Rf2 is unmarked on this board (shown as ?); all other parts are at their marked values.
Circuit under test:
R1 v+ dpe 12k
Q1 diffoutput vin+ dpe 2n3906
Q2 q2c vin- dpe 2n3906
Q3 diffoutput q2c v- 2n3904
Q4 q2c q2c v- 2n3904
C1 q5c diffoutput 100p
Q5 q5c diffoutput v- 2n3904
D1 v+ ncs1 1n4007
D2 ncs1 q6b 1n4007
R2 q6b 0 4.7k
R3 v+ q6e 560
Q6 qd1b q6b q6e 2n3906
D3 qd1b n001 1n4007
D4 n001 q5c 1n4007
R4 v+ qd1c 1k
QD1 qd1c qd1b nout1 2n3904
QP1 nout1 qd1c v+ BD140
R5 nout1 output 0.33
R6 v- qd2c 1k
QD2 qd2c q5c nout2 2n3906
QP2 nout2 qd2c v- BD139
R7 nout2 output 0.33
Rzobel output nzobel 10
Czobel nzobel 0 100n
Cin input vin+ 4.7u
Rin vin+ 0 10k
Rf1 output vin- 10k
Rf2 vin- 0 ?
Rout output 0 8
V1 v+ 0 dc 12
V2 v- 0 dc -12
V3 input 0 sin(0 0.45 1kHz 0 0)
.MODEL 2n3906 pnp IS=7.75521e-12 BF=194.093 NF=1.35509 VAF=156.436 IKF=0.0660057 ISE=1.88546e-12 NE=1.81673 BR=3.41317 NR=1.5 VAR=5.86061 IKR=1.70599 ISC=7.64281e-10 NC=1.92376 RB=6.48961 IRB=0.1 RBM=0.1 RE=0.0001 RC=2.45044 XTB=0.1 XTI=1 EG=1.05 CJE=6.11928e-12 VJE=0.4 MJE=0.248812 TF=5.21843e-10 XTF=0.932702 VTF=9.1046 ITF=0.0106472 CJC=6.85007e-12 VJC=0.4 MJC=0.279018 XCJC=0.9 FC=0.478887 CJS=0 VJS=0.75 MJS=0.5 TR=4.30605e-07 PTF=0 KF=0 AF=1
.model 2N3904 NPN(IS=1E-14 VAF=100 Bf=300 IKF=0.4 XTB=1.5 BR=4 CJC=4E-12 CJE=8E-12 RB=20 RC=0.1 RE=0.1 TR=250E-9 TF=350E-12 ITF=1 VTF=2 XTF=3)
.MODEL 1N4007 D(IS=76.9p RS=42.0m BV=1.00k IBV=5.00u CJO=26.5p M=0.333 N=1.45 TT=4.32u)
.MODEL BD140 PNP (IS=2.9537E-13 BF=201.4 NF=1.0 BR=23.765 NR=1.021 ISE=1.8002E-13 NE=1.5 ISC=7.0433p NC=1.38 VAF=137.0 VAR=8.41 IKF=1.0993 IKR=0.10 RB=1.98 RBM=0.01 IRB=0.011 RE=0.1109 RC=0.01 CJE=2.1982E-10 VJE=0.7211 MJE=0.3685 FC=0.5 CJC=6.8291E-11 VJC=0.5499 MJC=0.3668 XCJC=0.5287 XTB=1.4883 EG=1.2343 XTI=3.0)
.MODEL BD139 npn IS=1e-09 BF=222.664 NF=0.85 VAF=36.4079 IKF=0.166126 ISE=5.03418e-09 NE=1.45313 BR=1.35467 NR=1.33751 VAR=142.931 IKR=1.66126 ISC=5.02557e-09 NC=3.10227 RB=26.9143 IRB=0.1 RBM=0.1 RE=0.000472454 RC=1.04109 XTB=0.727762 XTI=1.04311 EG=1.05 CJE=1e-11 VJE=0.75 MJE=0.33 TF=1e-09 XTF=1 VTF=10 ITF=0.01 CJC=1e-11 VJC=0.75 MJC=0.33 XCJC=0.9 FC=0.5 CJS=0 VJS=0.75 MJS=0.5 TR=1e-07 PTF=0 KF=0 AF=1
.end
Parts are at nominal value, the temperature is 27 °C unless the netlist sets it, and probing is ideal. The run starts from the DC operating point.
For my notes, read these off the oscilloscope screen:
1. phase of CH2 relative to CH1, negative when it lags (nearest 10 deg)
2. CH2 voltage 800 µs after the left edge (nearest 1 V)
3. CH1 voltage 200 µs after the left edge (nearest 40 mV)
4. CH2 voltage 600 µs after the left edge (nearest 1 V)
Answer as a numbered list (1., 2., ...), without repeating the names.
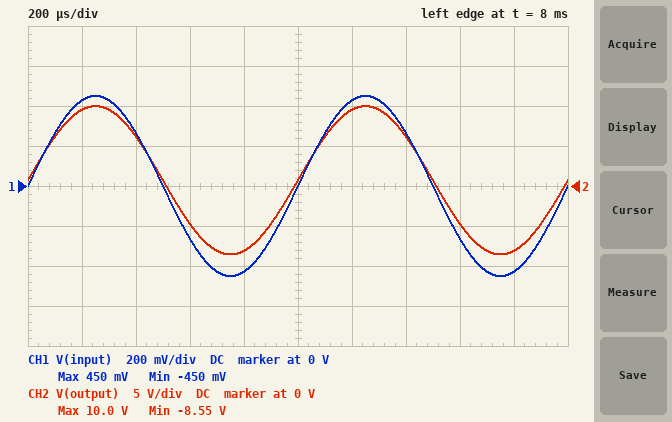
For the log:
1. 0 deg
2. -8 V
3. 440 mV
4. -5 V
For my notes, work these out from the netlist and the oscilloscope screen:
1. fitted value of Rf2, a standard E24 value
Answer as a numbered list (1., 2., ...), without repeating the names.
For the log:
1. 510 Ω
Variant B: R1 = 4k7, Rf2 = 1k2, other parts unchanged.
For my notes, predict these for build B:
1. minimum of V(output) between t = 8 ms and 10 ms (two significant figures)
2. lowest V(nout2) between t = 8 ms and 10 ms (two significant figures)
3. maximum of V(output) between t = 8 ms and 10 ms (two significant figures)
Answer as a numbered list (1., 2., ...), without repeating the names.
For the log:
1. -3.5 V
2. -3.6 V
3. 4.9 V
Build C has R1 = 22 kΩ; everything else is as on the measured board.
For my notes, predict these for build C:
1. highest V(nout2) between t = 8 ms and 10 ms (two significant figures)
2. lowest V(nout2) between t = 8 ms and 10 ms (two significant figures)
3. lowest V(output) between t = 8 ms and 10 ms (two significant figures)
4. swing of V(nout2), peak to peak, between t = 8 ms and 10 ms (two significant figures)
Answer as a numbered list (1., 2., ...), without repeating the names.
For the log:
1. 9.7 V
2. -9.2 V
3. -8.9 V
4. 19 V
